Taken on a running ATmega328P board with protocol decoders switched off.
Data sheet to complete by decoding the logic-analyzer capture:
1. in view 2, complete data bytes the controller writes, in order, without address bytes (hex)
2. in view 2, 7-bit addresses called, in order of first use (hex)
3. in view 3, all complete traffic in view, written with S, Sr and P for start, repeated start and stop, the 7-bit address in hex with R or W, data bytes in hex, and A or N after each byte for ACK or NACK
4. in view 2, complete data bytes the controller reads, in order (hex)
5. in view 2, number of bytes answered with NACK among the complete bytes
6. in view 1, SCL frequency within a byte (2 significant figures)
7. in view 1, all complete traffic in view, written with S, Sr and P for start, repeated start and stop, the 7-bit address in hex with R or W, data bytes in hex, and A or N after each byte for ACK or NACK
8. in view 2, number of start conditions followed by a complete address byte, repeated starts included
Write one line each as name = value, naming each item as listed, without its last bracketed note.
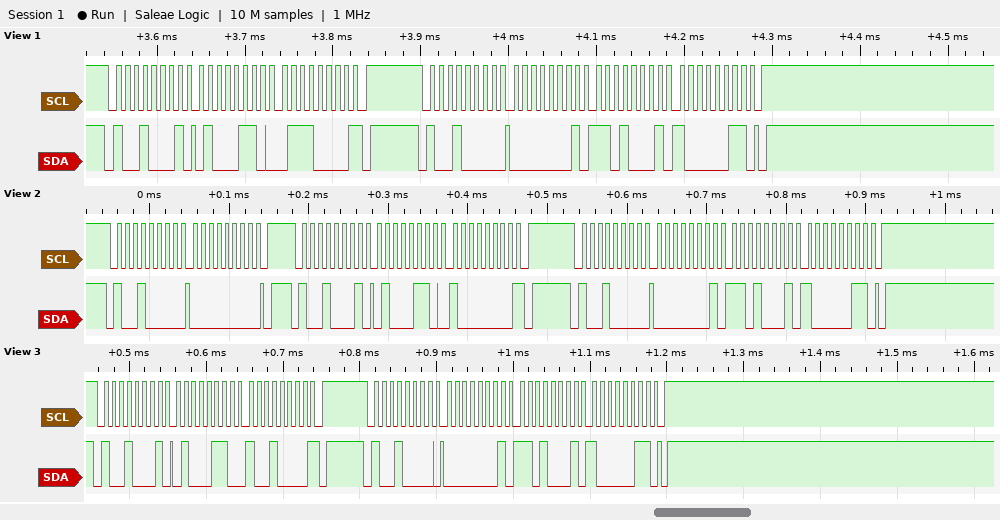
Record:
in view 2, complete data bytes the controller writes, in order, without address bytes = 00 01 D1 83
in view 2, 7-bit addresses called, in order of first use = 0x48
in view 3, all complete traffic in view, written with S, Sr and P for start, repeated start and stop, the 7-bit address in hex with R or W, data bytes in hex, and A or N after each byte for ACK or NACK = S 48R A 46 A 90 N P S 48W A 01 A D1 A 83 A P
in view 2, complete data bytes the controller reads, in order = 46 80
in view 2, number of bytes answered with NACK among the complete bytes = 1
in view 1, SCL frequency within a byte = 100 kHz
in view 1, all complete traffic in view, written with S, Sr and P for start, repeated start and stop, the 7-bit address in hex with R or W, data bytes in hex, and A or N after each byte for ACK or NACK = S 48R A 46 A 70 N P S 48W A 01 A D1 A 83 A P
in view 2, number of start conditions followed by a complete address byte, repeated starts included = 3
